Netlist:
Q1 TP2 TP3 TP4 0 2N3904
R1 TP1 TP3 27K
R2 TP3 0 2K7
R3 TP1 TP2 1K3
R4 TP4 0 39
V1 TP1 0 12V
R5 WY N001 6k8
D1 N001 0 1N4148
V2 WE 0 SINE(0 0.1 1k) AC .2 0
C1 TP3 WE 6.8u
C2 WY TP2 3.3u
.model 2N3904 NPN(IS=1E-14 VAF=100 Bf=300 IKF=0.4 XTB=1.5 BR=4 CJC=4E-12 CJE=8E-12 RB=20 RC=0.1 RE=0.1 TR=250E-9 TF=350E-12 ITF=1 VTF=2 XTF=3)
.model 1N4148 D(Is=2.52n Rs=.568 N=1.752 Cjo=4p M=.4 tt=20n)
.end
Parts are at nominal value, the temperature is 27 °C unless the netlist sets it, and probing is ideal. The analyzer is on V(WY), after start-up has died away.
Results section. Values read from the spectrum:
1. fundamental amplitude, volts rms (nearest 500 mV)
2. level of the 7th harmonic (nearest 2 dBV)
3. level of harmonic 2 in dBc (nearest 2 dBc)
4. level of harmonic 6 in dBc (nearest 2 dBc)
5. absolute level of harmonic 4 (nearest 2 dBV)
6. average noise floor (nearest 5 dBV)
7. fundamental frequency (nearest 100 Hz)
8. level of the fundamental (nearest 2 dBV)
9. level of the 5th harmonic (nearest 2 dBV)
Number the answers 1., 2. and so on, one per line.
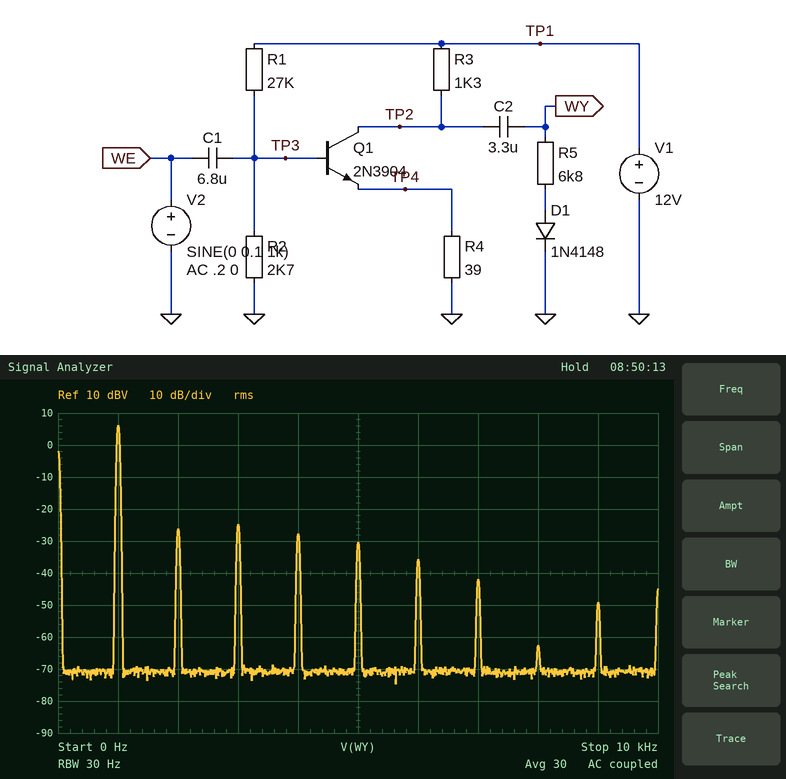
1. 2.0 V
2. -42 dBV
3. -32 dBc
4. -42 dBc
5. -28 dBV
6. -70 dBV
7. 1.0 kHz
8. 6 dBV
9. -30 dBV
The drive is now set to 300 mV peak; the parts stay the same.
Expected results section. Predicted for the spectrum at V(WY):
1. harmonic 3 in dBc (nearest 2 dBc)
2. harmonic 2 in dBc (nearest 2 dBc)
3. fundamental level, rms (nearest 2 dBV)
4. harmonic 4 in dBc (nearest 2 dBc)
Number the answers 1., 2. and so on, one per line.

1. -20 dBc
2. -18 dBc
3. 14 dBV
4. -32 dBc
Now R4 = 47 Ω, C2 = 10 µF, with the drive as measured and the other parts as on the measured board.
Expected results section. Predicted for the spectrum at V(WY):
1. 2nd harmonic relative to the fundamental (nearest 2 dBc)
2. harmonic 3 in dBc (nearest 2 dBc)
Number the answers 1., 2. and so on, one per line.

1. -42 dBc
2. -44 dBc
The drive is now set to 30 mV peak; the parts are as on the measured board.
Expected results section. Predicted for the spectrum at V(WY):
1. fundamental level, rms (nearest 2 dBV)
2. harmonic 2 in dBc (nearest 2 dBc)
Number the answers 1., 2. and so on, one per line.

1. -4 dBV
2. -52 dBc
